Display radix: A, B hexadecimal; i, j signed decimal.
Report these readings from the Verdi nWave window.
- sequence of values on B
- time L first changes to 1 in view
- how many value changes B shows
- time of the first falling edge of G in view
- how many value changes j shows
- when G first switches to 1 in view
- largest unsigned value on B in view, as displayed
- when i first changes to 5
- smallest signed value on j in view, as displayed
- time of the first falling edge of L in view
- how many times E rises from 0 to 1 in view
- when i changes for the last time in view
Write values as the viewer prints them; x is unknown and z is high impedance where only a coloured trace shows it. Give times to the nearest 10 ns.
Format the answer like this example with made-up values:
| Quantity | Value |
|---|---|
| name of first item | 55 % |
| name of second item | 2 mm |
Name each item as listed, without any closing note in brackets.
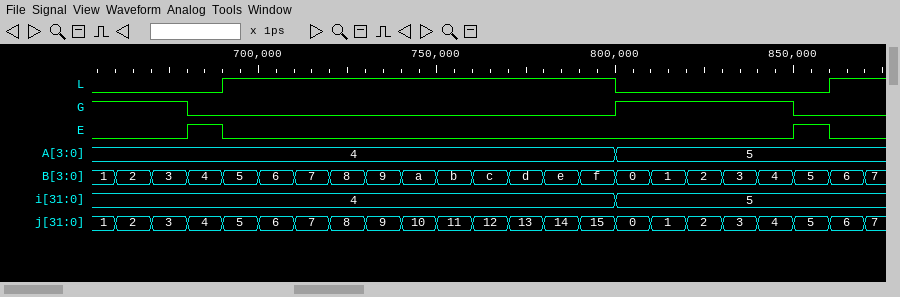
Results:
| Quantity | Value |
|---|---|
| sequence of values on B | 1, 2, 3, 4, 5, 6, 7, 8, 9, a, b, c, d, e, f, 0, 1, 2, 3, 4, 5, 6, 7 |
| time L first changes to 1 in view | 690 ns |
| how many value changes B shows | 22 |
| time of the first falling edge of G in view | 680 ns |
| how many value changes j shows | 22 |
| when G first switches to 1 in view | 800 ns |
| largest unsigned value on B in view, as displayed | f |
| when i first changes to 5 | 800 ns |
| smallest signed value on j in view, as displayed | 0 |
| time of the first falling edge of L in view | 800 ns |
| how many times E rises from 0 to 1 in view | 2 |
| when i changes for the last time in view | 800 ns |
